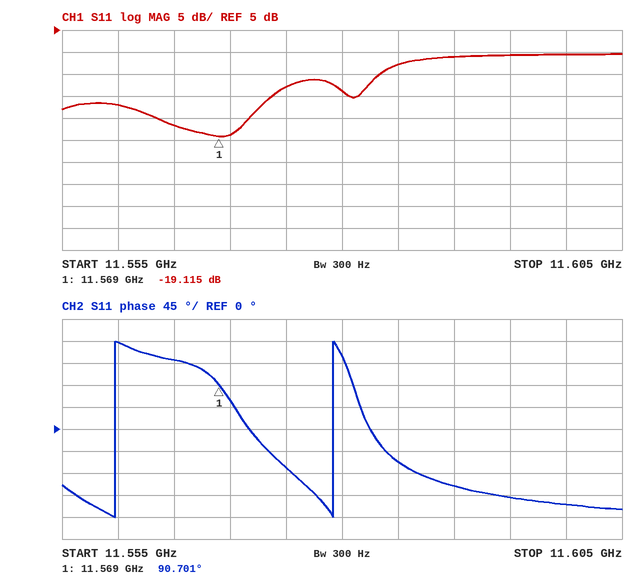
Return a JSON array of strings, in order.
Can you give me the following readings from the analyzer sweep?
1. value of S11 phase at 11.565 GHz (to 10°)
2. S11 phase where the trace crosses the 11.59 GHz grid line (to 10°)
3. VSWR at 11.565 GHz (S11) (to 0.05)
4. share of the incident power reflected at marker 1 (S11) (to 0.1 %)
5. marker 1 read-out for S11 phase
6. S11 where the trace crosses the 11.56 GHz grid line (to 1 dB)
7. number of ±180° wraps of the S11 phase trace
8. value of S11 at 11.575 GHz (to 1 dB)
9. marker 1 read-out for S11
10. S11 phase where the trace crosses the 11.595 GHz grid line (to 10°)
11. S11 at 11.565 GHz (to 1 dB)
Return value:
["140°", "-120°", "1.35", "1.2 %", "90.701°", "-12 dB", "2", "-8 dB", "-19.115 dB", "-140°", "-17 dB"]
